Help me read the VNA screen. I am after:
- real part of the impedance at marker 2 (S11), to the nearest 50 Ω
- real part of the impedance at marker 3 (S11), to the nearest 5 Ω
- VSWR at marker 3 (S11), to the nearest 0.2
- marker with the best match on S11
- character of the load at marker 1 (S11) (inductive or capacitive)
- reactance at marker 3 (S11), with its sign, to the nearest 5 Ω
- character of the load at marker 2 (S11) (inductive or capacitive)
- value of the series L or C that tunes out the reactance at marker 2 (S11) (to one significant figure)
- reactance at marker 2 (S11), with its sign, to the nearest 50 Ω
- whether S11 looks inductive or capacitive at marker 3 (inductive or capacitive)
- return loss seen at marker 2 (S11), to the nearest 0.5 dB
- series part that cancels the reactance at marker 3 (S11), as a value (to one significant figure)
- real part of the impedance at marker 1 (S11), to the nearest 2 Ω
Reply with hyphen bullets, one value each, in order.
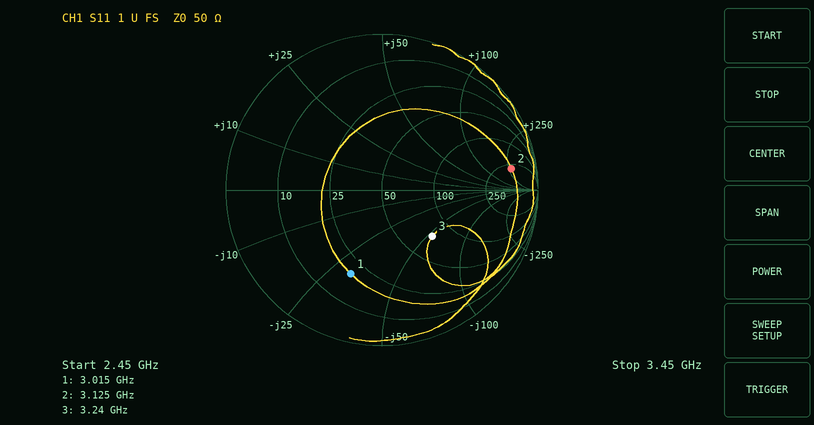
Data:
- 300 Ω
- 75 Ω
- 2.6
- marker 3
- capacitive
- -55 Ω
- inductive
- 200 fF
- +300 Ω
- capacitive
- 1.5 dB
- 3 nH
- 20 Ω
